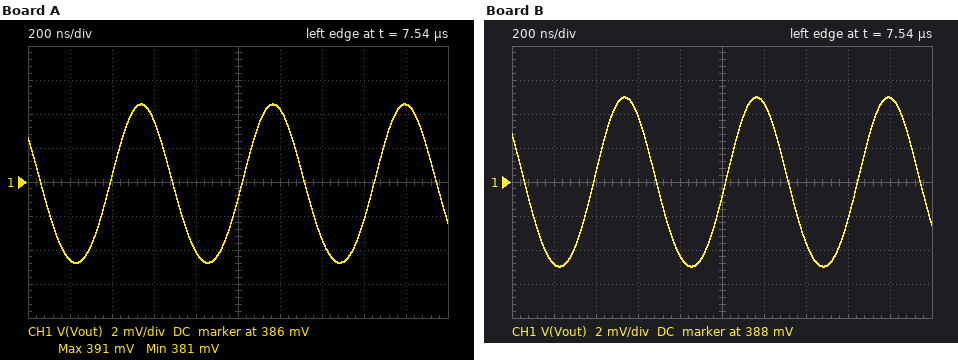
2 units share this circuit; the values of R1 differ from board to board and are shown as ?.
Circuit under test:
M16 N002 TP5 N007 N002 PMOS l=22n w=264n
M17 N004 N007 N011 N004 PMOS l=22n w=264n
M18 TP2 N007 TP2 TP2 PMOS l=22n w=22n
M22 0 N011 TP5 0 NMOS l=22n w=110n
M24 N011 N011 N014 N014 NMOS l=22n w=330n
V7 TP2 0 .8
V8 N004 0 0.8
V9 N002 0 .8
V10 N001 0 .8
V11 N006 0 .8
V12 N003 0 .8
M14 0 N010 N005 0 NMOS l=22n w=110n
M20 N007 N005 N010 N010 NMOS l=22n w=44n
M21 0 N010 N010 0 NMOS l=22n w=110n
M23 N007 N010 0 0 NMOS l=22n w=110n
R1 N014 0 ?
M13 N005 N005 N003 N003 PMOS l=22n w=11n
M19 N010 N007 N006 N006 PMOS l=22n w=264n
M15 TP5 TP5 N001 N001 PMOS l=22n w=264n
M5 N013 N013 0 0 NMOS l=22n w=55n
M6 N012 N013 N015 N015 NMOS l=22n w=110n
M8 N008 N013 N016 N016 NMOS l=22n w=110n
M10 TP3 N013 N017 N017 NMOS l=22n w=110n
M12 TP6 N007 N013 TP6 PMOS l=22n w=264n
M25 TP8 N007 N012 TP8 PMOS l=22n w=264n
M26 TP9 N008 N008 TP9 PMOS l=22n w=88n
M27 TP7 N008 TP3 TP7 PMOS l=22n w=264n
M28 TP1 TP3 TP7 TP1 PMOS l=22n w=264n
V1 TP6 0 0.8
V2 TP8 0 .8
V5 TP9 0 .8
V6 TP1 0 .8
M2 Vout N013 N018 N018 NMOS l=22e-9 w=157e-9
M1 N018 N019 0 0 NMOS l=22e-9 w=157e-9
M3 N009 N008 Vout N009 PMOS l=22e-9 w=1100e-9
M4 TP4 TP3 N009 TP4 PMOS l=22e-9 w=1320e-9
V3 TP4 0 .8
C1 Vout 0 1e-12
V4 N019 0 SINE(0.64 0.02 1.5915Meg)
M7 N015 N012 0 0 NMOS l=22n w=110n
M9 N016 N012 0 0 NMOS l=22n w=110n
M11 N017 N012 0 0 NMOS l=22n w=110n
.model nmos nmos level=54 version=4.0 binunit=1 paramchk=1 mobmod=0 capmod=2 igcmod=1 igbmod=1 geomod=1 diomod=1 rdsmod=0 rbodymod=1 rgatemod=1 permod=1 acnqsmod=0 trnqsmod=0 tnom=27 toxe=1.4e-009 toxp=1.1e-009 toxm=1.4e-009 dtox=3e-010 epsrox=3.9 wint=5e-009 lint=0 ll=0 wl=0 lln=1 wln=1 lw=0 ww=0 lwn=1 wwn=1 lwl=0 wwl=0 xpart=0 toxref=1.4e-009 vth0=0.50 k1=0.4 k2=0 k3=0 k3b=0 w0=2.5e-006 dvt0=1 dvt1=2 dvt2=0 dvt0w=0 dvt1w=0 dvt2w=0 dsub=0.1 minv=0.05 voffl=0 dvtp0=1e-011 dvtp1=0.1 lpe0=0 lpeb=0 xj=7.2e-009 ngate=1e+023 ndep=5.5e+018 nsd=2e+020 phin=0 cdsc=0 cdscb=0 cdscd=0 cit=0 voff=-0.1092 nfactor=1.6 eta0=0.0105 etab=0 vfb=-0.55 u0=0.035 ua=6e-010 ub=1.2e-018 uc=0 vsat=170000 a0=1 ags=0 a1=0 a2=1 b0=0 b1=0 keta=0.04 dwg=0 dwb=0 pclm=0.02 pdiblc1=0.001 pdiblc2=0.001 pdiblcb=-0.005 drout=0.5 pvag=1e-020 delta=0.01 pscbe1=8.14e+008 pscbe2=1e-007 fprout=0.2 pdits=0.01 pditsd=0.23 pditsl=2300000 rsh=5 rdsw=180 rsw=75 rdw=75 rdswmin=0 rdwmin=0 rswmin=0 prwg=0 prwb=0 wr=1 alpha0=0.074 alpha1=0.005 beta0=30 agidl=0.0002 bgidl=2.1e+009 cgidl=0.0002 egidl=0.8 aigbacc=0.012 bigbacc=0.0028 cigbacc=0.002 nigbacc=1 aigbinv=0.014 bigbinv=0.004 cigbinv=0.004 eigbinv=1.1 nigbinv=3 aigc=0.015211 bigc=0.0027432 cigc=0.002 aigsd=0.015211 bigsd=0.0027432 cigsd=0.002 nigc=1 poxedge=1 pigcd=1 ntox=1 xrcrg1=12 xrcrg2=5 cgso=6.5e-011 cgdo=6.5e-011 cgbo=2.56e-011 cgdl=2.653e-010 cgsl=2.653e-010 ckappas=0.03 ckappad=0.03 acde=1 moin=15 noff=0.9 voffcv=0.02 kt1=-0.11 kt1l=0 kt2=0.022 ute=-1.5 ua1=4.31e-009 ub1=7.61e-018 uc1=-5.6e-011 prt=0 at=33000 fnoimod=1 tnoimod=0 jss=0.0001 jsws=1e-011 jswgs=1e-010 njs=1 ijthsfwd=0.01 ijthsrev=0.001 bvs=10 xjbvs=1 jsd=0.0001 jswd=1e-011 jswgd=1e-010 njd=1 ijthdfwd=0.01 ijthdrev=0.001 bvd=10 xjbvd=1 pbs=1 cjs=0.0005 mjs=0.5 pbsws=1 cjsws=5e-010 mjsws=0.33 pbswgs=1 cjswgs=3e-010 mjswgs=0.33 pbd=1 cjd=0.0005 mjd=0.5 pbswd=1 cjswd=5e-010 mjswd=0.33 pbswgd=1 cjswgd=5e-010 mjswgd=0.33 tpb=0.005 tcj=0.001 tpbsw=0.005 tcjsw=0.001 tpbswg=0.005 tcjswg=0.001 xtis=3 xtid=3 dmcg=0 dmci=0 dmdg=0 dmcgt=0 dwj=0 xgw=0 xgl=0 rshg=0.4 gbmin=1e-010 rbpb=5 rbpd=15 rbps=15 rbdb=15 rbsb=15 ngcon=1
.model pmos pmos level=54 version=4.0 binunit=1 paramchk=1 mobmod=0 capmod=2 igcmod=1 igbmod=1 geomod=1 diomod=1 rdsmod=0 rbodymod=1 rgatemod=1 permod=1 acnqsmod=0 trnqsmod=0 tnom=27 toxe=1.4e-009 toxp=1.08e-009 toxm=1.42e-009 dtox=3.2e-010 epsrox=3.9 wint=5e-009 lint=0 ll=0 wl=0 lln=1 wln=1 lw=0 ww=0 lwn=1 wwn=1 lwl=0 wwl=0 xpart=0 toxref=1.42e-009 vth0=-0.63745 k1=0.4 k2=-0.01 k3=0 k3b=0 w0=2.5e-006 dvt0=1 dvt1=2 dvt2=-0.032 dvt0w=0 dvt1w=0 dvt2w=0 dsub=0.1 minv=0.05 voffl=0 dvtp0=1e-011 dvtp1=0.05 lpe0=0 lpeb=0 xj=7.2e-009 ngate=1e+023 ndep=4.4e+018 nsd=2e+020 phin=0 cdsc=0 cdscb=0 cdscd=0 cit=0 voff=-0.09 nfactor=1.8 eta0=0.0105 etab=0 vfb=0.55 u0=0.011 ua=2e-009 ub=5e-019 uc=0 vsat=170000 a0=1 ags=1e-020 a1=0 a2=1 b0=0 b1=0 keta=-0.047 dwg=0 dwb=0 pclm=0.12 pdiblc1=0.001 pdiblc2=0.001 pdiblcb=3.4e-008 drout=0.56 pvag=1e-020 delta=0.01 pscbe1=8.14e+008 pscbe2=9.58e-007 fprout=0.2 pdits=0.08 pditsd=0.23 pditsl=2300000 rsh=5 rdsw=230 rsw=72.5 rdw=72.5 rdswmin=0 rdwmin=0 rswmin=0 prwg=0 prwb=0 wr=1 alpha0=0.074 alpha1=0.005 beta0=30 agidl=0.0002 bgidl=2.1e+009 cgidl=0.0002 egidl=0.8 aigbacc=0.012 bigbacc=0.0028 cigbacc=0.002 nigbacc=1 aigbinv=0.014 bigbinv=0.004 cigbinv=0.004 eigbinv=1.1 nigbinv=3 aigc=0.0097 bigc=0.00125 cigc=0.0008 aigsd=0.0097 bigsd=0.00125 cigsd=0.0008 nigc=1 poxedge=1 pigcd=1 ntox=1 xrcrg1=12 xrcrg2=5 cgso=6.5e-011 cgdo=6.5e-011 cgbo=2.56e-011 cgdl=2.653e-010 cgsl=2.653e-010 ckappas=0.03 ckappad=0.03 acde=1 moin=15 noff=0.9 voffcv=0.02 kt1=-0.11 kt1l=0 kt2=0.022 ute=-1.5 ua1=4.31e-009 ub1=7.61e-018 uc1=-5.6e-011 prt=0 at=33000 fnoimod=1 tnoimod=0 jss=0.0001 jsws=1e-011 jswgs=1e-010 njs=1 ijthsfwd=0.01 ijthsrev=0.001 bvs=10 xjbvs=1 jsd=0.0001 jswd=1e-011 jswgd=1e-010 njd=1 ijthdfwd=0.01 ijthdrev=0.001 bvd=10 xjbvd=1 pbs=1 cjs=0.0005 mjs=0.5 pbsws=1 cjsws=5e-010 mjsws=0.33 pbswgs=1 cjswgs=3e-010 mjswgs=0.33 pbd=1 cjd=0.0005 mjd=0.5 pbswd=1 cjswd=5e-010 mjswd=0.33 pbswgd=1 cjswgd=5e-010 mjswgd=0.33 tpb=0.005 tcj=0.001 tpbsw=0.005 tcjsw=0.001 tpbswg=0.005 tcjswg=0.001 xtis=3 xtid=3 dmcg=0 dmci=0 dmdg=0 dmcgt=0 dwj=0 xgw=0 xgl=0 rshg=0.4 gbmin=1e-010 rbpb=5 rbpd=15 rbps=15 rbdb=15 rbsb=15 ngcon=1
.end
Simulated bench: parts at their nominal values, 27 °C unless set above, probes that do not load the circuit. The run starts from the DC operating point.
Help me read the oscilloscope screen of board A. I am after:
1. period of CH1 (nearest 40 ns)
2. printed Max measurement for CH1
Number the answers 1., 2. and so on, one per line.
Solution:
1. 640 ns
2. 391 mV
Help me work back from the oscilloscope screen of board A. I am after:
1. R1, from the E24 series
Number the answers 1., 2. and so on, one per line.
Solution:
1. 12 kΩ
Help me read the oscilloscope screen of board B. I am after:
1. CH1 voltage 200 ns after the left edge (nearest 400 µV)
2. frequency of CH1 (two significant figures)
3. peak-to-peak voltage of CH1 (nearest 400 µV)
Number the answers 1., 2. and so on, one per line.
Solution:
1. 383.2 mV
2. 1.6 MHz
3. 10.0 mV
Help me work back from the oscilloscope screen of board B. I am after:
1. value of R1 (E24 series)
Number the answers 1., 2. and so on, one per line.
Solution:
1. 11 kΩ
